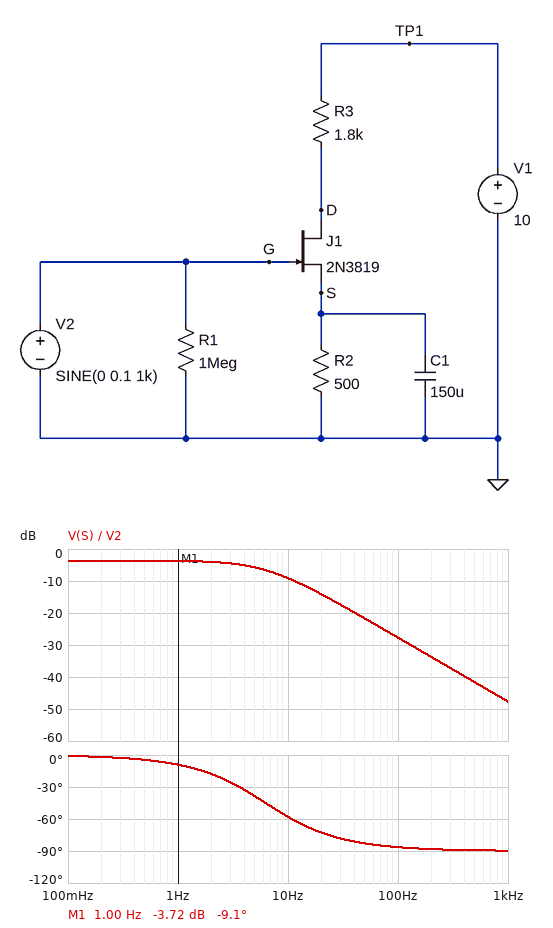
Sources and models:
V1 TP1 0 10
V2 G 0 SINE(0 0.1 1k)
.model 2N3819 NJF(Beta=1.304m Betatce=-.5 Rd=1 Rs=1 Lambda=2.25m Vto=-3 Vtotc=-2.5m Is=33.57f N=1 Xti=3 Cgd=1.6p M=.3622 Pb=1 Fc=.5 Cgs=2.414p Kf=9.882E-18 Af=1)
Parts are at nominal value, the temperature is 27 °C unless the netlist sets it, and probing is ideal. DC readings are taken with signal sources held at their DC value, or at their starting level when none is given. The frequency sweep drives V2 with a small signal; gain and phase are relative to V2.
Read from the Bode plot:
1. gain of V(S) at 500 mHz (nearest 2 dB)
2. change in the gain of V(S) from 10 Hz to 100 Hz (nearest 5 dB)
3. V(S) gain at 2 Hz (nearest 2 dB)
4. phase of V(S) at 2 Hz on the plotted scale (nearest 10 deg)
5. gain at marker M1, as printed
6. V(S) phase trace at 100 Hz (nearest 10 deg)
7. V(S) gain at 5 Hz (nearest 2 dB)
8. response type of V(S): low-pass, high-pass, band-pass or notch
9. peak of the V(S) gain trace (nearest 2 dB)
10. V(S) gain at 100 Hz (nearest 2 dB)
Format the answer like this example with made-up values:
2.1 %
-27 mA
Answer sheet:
-4 dB
-20 dB
-4 dB
-20 deg
-3.72 dB
-90 deg
-6 dB
low-pass
-4 dB
-28 dB
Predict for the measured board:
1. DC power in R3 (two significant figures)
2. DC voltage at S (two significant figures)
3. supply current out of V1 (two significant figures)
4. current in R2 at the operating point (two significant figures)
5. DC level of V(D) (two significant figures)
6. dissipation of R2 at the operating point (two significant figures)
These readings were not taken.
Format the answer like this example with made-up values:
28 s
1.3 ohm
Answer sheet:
16 mW
1.5 V
3.0 mA
3.0 mA
4.6 V
4.4 mW
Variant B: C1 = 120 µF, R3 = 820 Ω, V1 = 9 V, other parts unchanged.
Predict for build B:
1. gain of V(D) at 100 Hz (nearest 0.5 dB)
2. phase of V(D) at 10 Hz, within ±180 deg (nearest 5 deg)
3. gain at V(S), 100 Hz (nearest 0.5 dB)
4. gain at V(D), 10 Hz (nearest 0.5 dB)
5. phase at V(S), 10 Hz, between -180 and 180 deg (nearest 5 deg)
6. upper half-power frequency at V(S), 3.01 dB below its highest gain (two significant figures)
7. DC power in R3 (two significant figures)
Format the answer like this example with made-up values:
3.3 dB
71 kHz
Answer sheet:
10.0 dB
-155 deg
-25.5 dB
8.5 dB
-50 deg
7.9 Hz
7.3 mW
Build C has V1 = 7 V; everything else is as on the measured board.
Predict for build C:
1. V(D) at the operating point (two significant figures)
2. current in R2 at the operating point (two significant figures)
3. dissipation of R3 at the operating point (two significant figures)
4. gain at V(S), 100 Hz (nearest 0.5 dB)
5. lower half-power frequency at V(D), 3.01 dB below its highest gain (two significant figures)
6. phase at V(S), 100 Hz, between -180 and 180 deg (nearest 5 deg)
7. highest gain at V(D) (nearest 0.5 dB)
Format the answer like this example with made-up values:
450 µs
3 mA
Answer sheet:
2.2 V
2.7 mA
13 mW
-46.5 dB
580 mHz
-90 deg
-2.0 dB
